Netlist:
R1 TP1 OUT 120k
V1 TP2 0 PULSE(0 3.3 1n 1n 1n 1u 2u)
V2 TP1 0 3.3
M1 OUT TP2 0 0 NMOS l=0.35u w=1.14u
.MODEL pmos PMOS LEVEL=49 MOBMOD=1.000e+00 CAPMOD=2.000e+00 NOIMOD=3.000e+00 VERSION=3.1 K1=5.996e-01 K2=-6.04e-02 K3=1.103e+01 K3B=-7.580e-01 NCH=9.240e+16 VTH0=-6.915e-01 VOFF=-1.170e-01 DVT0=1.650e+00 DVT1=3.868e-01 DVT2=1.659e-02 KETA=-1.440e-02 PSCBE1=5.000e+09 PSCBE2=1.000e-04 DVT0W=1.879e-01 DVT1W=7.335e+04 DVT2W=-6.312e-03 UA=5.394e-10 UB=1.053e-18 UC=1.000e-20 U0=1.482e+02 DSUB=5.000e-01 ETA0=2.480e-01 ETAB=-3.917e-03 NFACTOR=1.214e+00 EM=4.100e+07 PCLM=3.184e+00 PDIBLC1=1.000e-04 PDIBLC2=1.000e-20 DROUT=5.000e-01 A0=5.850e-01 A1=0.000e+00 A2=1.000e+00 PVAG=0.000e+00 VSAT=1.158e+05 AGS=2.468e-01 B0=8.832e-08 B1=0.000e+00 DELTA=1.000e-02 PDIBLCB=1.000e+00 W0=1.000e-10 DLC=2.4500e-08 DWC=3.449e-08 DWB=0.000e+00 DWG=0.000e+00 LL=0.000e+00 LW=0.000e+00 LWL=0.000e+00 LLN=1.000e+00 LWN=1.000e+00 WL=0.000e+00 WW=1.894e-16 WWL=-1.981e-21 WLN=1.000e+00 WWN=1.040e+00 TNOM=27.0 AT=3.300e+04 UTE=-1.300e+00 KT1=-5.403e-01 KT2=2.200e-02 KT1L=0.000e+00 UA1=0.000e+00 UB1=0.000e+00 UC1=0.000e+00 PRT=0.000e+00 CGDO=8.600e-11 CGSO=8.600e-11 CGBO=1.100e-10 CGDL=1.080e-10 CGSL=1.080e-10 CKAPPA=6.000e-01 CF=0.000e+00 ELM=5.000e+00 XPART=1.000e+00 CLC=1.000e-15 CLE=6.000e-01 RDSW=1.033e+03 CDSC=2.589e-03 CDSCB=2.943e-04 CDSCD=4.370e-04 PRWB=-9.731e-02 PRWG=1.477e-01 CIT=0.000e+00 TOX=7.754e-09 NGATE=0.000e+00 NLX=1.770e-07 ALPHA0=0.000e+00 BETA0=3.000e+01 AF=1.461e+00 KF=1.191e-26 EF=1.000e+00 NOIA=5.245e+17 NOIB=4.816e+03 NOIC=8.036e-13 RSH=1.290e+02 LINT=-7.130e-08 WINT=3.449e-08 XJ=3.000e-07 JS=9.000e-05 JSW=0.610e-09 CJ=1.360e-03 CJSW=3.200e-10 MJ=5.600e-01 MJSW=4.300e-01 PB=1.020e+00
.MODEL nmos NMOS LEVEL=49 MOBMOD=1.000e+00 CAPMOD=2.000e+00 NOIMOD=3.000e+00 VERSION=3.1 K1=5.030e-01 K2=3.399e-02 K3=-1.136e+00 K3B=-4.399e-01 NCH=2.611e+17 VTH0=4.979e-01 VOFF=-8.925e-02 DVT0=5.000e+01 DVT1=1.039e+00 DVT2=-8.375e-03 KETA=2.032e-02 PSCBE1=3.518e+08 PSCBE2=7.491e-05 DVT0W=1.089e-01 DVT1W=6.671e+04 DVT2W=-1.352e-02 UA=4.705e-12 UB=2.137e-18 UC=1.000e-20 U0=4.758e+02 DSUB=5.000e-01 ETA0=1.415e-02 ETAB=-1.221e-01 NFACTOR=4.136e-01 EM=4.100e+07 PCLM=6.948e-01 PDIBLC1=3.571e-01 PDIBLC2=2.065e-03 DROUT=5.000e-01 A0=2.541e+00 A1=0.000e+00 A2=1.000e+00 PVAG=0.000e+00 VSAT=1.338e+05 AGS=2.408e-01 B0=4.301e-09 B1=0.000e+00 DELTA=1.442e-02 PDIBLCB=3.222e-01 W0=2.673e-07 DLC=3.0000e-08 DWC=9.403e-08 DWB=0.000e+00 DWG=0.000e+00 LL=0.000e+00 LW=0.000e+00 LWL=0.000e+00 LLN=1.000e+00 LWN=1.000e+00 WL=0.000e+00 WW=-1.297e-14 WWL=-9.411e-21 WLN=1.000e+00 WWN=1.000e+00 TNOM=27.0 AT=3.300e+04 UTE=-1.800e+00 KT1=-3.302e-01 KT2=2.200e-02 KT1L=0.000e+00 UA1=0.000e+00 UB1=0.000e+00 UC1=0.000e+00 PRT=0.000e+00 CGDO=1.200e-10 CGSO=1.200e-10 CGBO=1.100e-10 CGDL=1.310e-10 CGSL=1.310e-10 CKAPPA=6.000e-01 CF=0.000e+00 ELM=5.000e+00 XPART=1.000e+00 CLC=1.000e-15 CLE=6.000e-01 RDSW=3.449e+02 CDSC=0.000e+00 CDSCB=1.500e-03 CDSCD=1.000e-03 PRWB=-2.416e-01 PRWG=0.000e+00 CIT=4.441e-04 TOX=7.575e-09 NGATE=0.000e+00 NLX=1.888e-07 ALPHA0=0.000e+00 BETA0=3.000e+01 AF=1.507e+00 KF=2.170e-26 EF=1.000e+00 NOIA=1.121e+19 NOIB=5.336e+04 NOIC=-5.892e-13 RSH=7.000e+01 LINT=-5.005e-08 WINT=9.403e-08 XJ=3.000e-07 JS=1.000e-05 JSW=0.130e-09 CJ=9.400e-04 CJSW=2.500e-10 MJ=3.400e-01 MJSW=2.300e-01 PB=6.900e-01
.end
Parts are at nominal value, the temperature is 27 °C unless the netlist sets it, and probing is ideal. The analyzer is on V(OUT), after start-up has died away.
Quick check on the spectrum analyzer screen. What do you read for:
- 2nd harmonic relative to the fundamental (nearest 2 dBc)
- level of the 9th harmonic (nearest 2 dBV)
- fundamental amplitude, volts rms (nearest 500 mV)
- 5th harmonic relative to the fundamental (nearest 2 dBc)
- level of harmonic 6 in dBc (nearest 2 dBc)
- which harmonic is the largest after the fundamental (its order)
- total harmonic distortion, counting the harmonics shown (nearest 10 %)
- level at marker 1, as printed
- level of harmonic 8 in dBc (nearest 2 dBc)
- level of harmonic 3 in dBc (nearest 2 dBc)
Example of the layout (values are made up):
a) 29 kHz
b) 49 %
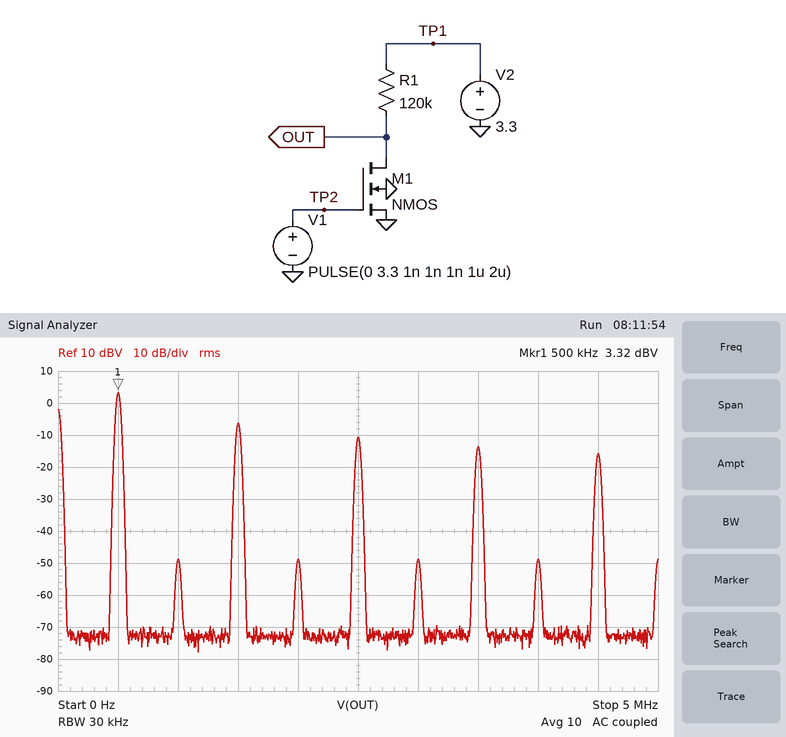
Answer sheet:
a) -52 dBc
b) -16 dBV
c) 1.5 V
d) -14 dBc
e) -52 dBc
f) 3
g) 40 %
h) 3.32 dBV
i) -52 dBc
j) -10 dBc
